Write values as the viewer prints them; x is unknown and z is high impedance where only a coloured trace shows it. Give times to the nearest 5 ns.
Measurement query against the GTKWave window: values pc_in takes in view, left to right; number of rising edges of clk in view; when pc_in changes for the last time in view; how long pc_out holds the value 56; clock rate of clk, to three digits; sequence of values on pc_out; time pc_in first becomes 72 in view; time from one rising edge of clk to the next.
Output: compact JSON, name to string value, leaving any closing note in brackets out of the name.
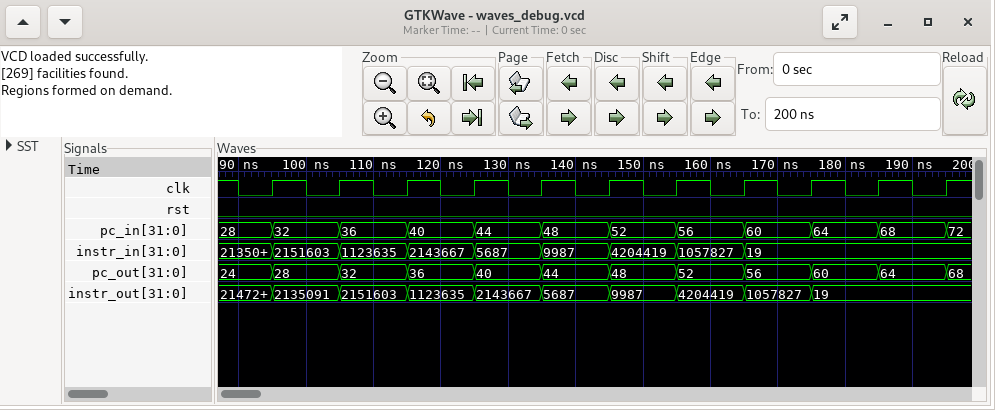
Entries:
{"values pc_in takes in view, left to right": "28, 32, 36, 40, 44, 48, 52, 56, 60, 64, 68, 72", "number of rising edges of clk in view": "11", "when pc_in changes for the last time in view": "195 ns", "how long pc_out holds the value 56": "10 ns", "clock rate of clk, to three digits": "100 MHz", "sequence of values on pc_out": "24, 28, 32, 36, 40, 44, 48, 52, 56, 60, 64, 68", "time pc_in first becomes 72 in view": "195 ns", "time from one rising edge of clk to the next": "10 ns"}
